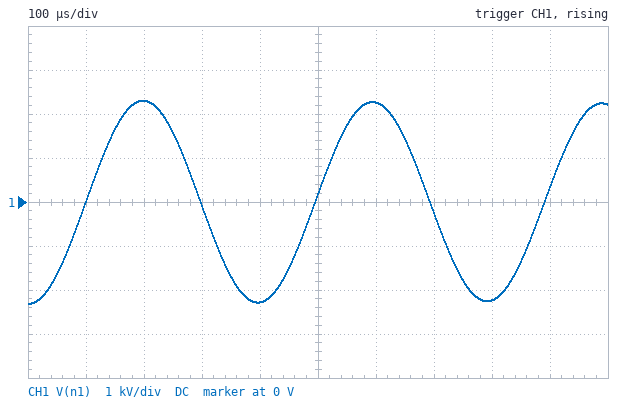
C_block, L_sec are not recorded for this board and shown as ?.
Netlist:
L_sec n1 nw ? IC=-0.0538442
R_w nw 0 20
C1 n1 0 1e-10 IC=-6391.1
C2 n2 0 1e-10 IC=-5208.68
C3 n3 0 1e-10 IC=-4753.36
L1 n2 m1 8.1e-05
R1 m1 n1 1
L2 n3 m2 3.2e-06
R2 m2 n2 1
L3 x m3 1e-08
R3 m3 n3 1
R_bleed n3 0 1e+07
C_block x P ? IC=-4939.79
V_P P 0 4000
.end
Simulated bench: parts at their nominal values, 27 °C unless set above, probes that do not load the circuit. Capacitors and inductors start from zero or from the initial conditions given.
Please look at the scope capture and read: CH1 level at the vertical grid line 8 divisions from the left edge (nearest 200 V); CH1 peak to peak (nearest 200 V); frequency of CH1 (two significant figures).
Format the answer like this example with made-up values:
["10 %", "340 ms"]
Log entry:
["-2.2 kV", "4.6 kV", "2.5 kHz"]
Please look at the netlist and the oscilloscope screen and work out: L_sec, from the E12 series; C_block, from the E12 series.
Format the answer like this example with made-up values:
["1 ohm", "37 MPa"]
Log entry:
["2.2 H", "1.5 nF"]
